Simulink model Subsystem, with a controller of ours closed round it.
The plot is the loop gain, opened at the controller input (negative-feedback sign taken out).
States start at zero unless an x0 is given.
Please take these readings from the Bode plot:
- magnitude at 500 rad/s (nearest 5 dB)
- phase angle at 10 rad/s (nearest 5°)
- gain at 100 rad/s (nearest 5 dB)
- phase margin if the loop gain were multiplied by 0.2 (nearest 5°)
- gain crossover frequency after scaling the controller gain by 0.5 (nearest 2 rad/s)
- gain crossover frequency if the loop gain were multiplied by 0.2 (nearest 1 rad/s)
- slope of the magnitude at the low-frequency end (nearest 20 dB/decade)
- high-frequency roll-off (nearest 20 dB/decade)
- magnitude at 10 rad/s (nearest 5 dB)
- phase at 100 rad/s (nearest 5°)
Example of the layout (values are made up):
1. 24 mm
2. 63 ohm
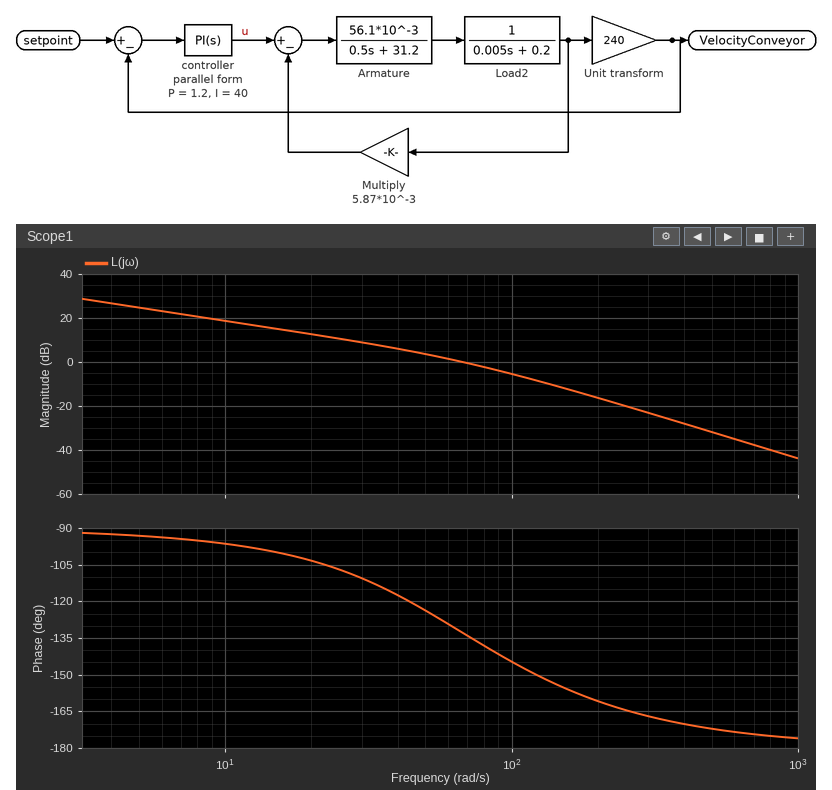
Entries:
1. -30 dB
2. -95°
3. -5 dB
4. 80°
5. 40 rad/s
6. 17 rad/s
7. -20 dB/decade
8. -40 dB/decade
9. 20 dB
10. -145°
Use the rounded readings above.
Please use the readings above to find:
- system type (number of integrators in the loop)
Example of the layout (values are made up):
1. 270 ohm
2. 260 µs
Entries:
1. 1
